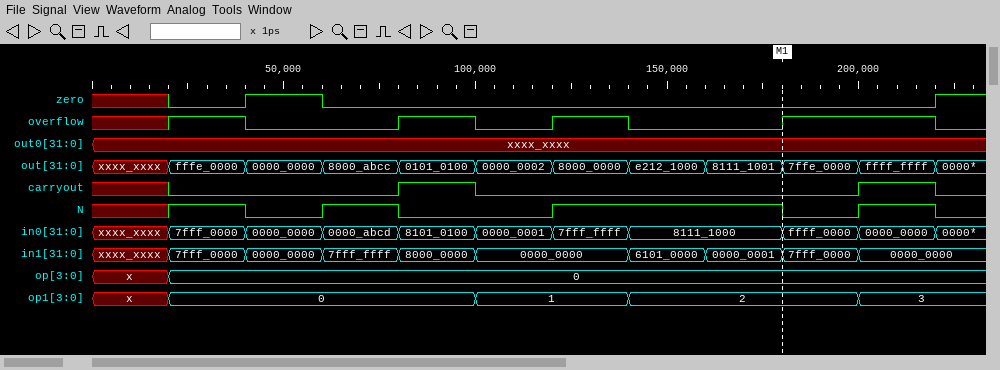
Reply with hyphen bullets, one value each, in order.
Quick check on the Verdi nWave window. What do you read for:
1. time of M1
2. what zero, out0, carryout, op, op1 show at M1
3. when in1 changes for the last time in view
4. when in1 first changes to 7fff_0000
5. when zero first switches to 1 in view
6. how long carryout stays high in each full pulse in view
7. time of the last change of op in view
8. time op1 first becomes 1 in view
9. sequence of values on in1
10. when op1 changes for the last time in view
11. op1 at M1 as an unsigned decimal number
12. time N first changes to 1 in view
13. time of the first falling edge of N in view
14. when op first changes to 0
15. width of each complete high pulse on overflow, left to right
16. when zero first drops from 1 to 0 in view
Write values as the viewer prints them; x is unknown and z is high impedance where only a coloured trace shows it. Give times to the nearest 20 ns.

- 180 ns
- zero=0, out0=xxxx_xxxx, carryout=0, op=0, op1=2
- 200 ns
- 20 ns
- 40 ns
- 20 ns, 20 ns
- 20 ns
- 100 ns
- xxxx_xxxx, 7fff_0000, 0000_0000, 7fff_ffff, 8000_0000, 0000_0000, 6101_0000, 0000_0001, 7fff_0000, 0000_0000
- 200 ns
- 2
- 20 ns
- 40 ns
- 20 ns
- 20 ns, 20 ns, 40 ns
- 60 ns
